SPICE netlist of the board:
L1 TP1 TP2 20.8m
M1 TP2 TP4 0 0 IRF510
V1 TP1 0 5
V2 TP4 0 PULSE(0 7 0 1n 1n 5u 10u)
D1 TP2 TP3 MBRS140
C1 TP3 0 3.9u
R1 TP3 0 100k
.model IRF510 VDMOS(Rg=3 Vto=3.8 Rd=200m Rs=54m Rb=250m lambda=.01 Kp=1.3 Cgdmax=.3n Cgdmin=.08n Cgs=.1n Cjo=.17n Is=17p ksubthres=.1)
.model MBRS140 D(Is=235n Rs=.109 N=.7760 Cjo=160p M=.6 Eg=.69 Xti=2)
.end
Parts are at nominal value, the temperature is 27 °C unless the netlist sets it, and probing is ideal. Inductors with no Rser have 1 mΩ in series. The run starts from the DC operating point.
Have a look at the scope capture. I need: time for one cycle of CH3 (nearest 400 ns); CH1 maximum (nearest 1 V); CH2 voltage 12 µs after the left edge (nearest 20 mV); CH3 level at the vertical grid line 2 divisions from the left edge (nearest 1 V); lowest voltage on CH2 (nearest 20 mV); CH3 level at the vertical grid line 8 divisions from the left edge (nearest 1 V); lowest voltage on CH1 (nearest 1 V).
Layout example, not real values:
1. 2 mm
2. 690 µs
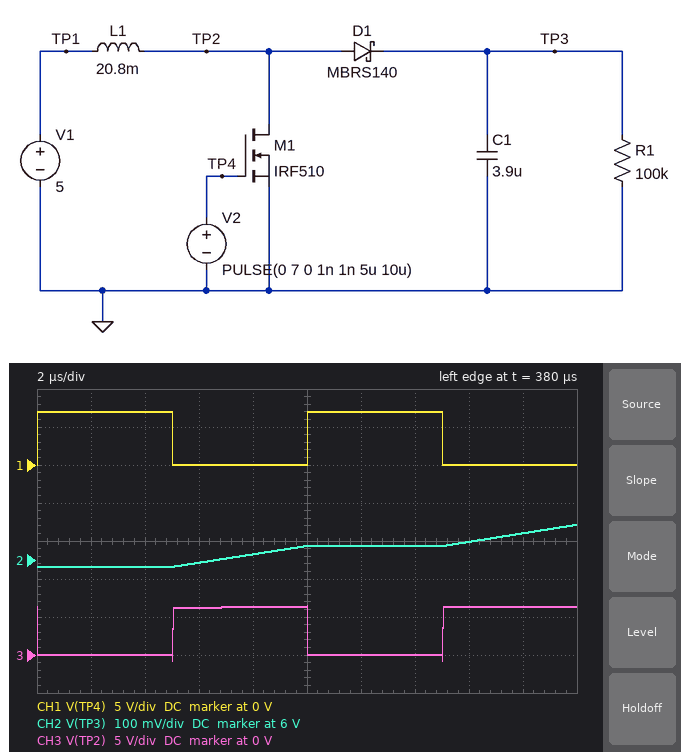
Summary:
1. 10.0 µs
2. 7 V
3. 6.04 V
4. 0 V
5. 5.98 V
6. 6 V
7. 0 V
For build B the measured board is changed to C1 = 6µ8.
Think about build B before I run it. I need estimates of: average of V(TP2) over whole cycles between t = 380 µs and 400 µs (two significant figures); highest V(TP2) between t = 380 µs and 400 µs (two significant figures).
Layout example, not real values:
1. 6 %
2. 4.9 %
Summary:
1. 2.9 V
2. 6.0 V
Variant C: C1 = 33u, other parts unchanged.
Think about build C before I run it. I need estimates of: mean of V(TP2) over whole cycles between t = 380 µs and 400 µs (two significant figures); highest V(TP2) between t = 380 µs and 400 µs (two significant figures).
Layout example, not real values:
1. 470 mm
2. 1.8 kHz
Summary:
1. 2.6 V
2. 5.4 V
